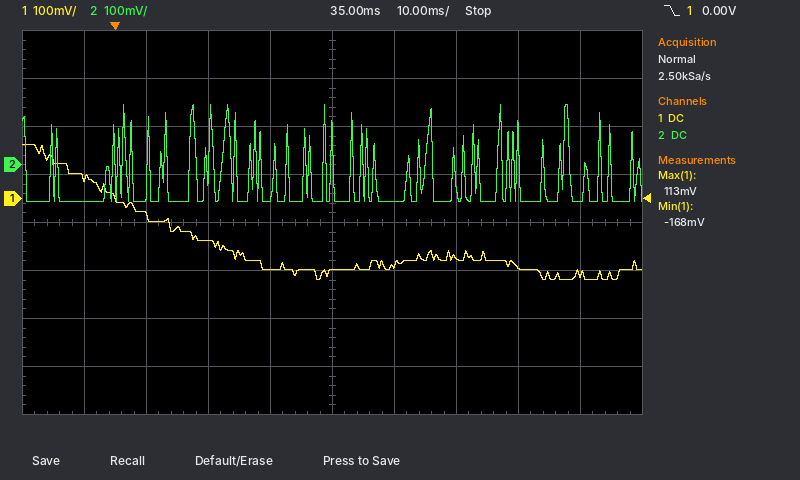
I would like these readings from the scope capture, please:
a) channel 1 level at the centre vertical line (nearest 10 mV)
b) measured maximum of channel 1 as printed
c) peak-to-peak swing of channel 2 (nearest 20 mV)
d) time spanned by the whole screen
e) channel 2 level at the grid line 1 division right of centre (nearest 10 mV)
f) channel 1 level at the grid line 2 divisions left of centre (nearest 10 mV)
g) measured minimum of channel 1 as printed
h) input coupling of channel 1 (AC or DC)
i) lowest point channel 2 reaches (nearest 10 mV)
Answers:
-150 mV
113 mV
200 mV
100 ms
-80 mV
-90 mV
-168 mV
DC
-80 mV
